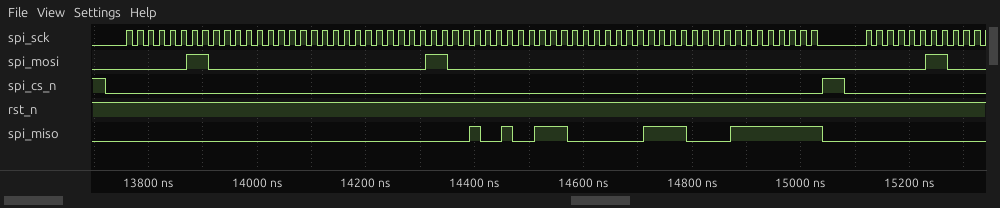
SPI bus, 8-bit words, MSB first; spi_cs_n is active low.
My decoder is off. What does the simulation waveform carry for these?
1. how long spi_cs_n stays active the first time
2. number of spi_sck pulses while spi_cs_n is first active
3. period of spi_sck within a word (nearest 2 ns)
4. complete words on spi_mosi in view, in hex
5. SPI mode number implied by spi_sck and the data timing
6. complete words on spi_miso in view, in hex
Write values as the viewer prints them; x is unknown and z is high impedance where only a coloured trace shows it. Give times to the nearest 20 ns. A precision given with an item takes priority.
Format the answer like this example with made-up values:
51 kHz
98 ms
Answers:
1320 ns
64
20 ns
03, 00, 00, 0C, 00, 00, 00, 00, 03
0
00, 00, 00, 00, 93, 80, F0, FF, 00
